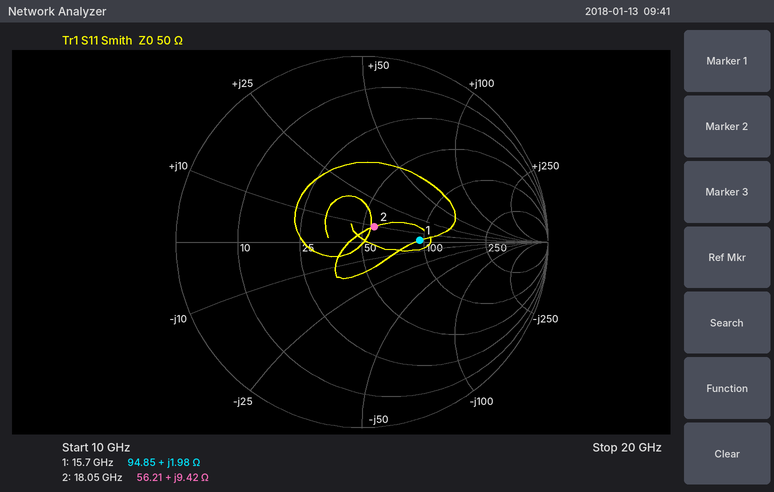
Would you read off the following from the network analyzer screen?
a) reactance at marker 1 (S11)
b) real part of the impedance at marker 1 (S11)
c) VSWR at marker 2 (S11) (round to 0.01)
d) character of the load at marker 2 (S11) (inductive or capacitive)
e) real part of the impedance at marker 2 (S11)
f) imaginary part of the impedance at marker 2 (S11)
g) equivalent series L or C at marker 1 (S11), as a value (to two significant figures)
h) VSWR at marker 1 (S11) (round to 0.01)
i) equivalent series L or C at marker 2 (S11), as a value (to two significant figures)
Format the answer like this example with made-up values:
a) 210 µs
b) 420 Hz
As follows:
a) +1.98 Ω
b) 94.85 Ω
c) 1.24
d) inductive
e) 56.21 Ω
f) +9.42 Ω
g) 20 pH
h) 1.90
i) 83 pH
